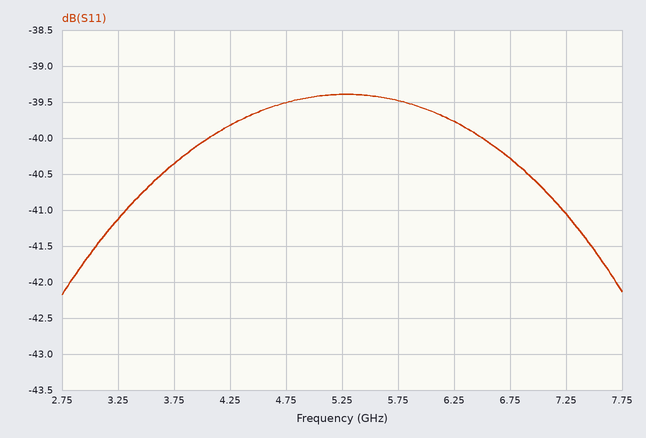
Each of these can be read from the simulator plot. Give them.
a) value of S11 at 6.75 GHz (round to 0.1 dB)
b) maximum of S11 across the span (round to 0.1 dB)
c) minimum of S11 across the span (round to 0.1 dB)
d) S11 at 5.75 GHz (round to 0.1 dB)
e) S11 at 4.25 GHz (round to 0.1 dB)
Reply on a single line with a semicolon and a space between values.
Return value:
-40.3 dB; -39.4 dB; -42.2 dB; -39.5 dB; -39.8 dB
